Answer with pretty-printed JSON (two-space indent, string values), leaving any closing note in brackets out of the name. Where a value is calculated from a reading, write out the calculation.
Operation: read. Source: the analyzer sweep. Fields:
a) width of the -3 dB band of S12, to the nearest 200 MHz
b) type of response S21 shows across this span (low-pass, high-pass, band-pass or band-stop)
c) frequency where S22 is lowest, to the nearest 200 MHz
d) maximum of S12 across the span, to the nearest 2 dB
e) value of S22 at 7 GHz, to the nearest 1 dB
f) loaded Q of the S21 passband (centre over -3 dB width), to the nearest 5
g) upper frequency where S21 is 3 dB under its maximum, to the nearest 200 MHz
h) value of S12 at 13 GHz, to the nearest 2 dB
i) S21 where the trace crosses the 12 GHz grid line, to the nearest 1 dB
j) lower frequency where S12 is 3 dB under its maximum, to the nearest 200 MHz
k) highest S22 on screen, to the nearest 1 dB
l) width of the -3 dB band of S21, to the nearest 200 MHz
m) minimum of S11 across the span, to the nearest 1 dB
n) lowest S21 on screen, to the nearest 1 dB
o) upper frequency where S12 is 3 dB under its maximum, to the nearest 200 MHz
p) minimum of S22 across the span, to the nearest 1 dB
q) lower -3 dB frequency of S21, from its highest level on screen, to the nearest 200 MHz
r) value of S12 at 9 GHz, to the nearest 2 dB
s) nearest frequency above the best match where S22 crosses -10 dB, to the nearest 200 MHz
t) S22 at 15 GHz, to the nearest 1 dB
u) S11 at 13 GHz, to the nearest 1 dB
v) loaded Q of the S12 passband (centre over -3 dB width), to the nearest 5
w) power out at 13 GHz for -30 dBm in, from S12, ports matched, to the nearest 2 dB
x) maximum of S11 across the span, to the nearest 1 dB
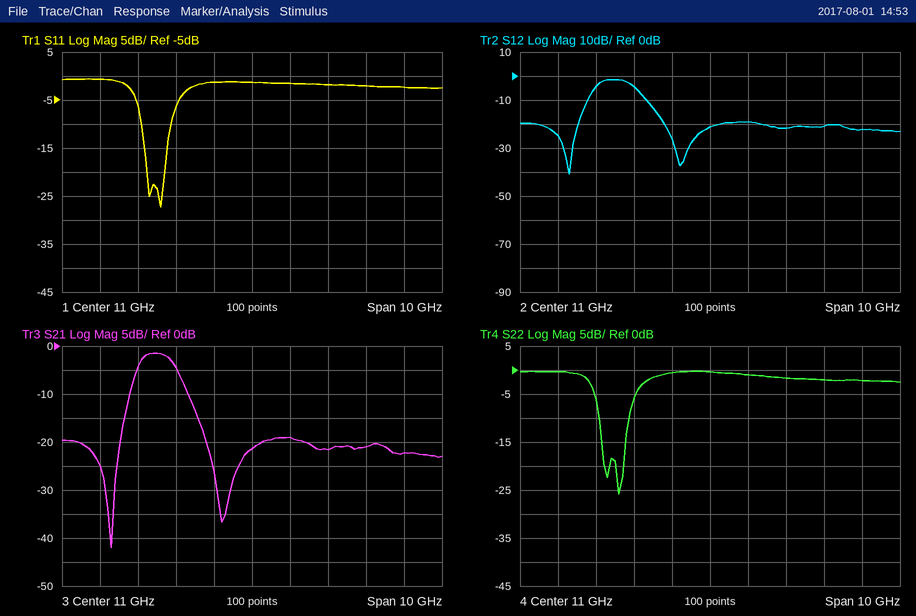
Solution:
{
  "width of the -3 dB band of S12, to the nearest 200 MHz": "9.0 GHz − 8.0 GHz = 1.0 GHz",
  "type of response S21 shows across this span": "band-pass",
  "frequency where S22 is lowest, to the nearest 200 MHz": "8.6 GHz",
  "maximum of S12 across the span, to the nearest 2 dB": "-2 dB",
  "value of S22 at 7 GHz, to the nearest 1 dB": "0 dB",
  "loaded Q of the S21 passband (centre over -3 dB width), to the nearest 5": "8.5 GHz / 1 GHz ≈ 8.50, so 10 to the nearest 5",
  "upper frequency where S21 is 3 dB under its maximum, to the nearest 200 MHz": "9.0 GHz",
  "value of S12 at 13 GHz, to the nearest 2 dB": "-22 dB",
  "S21 where the trace crosses the 12 GHz grid line, to the nearest 1 dB": "-19 dB",
  "lower frequency where S12 is 3 dB under its maximum, to the nearest 200 MHz": "8.0 GHz",
  "highest S22 on screen, to the nearest 1 dB": "0 dB",
  "width of the -3 dB band of S21, to the nearest 200 MHz": "9.0 GHz − 8.0 GHz = 1.0 GHz",
  "minimum of S11 across the span, to the nearest 1 dB": "-27 dB",
  "lowest S21 on screen, to the nearest 1 dB": "-42 dB",
  "upper frequency where S12 is 3 dB under its maximum, to the nearest 200 MHz": "9.0 GHz",
  "minimum of S22 across the span, to the nearest 1 dB": "-26 dB",
  "lower -3 dB frequency of S21, from its highest level on screen, to the nearest 200 MHz": "8.0 GHz",
  "value of S12 at 9 GHz, to the nearest 2 dB": "-4 dB",
  "nearest frequency above the best match where S22 crosses -10 dB, to the nearest 200 MHz": "8.8 GHz",
  "S22 at 15 GHz, to the nearest 1 dB": "-2 dB",
  "S11 at 13 GHz, to the nearest 1 dB": "-2 dB",
  "loaded Q of the S12 passband (centre over -3 dB width), to the nearest 5": "8.5 GHz / 1 GHz ≈ 8.50, so 10 to the nearest 5",
  "power out at 13 GHz for -30 dBm in, from S12, ports matched, to the nearest 2 dB": "-30 dBm + (-22 dB) = -52 dBm",
  "maximum of S11 across the span, to the nearest 1 dB": "-1 dB"
}
